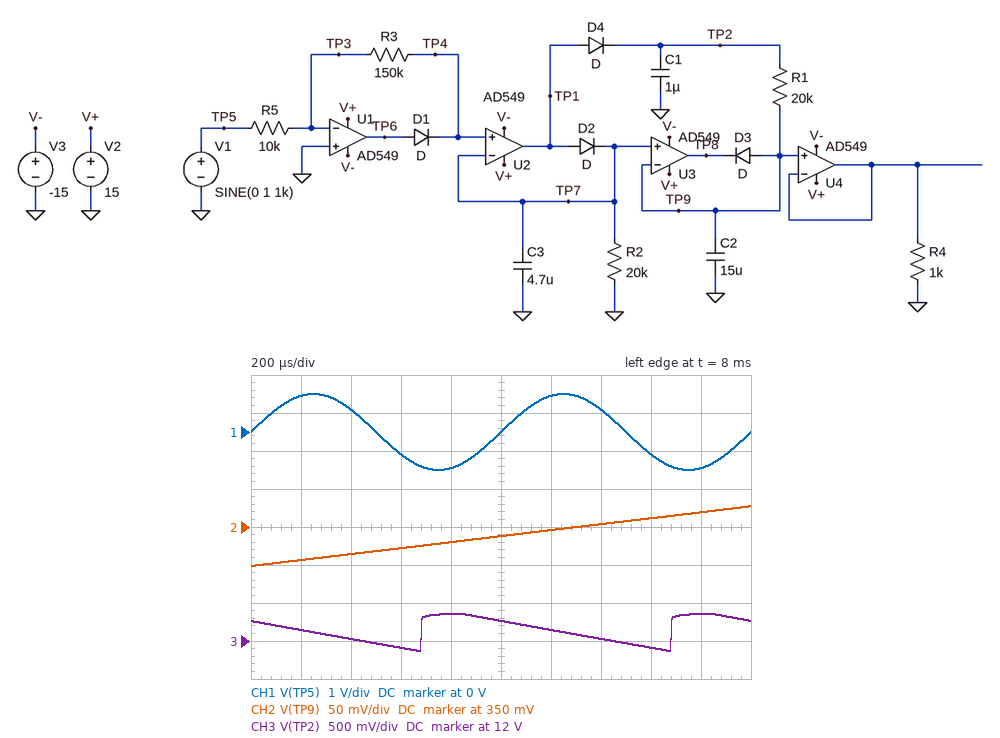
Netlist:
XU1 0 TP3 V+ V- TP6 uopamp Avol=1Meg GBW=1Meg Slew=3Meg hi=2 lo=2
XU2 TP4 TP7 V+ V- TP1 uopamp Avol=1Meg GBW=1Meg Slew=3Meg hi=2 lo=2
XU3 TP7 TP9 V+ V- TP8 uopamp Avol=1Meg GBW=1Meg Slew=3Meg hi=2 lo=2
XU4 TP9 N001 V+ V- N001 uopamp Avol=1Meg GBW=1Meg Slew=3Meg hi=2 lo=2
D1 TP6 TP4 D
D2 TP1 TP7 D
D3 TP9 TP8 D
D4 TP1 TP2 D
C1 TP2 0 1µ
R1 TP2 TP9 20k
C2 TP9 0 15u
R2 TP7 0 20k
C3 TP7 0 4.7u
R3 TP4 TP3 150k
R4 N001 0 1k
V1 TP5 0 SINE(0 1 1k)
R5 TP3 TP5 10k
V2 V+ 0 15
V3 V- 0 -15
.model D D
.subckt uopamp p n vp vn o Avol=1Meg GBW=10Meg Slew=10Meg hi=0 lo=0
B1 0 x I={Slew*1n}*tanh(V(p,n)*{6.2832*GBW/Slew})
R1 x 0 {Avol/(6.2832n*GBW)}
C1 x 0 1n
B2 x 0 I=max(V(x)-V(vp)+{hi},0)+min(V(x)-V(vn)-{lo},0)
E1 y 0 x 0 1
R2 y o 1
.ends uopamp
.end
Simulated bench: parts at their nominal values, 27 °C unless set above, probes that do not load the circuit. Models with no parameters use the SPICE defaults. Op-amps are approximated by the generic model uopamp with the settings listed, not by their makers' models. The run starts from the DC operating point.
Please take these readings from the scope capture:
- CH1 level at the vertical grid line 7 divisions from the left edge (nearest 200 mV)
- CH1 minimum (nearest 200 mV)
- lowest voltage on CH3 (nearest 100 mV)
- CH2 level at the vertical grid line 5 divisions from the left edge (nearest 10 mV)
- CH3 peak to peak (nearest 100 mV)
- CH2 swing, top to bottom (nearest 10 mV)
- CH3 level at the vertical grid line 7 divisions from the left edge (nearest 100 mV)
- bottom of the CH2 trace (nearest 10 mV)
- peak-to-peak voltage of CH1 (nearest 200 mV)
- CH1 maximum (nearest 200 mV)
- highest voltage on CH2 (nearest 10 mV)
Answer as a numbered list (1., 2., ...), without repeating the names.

1. 600 mV
2. -1.0 V
3. 11.9 V
4. 340 mV
5. 500 mV
6. 80 mV
7. 12.0 V
8. 300 mV
9. 2.0 V
10. 1.0 V
11. 380 mV
